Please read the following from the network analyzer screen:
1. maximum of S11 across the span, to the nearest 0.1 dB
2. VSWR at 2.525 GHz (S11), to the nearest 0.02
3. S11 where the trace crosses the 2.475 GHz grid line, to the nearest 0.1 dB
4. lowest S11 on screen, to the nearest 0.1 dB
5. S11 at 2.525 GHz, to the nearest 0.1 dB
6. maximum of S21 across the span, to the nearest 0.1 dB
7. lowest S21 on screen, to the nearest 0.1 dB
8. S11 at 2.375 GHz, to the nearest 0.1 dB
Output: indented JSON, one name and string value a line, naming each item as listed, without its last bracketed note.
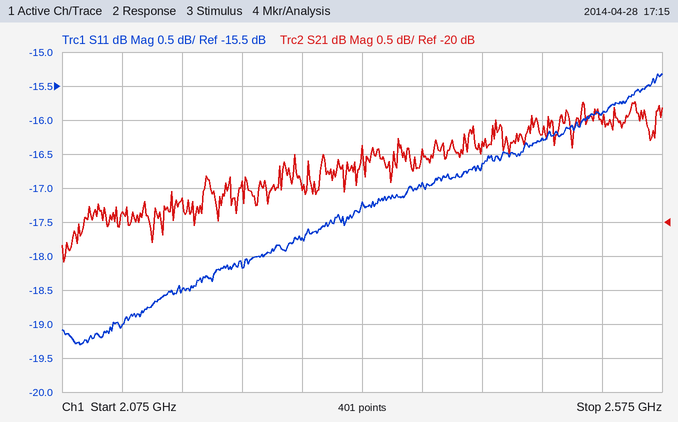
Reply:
{
  "maximum of S11 across the span, to the nearest 0.1 dB": "-15.3 dB",
  "VSWR at 2.525 GHz (S11), to the nearest 0.02": "1.38",
  "S11 where the trace crosses the 2.475 GHz grid line, to the nearest 0.1 dB": "-16.3 dB",
  "lowest S11 on screen, to the nearest 0.1 dB": "-19.3 dB",
  "S11 at 2.525 GHz, to the nearest 0.1 dB": "-15.9 dB",
  "maximum of S21 across the span, to the nearest 0.1 dB": "-18.2 dB",
  "lowest S21 on screen, to the nearest 0.1 dB": "-20.6 dB",
  "S11 at 2.375 GHz, to the nearest 0.1 dB": "-16.9 dB"
}
